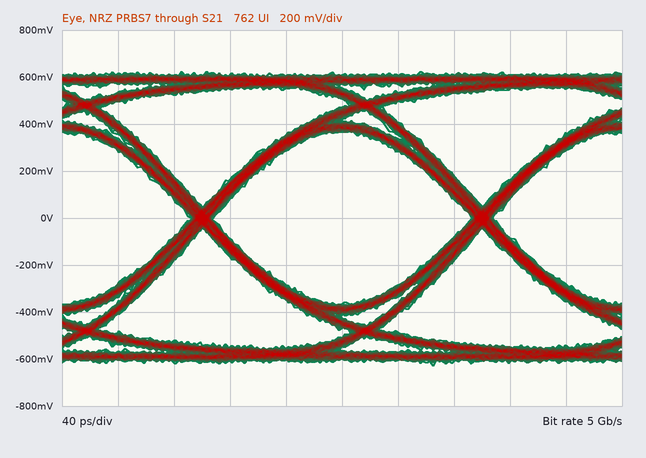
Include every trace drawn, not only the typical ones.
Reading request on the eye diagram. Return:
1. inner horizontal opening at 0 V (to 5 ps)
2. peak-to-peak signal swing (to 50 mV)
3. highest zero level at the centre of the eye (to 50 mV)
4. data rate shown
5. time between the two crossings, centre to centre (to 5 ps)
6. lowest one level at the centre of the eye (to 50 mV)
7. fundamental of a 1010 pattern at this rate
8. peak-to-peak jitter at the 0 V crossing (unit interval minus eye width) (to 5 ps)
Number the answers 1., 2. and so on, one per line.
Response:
1. 185 ps
2. 1.25 V
3. -350 mV
4. 5 Gb/s
5. 200 ps
6. 350 mV
7. 2.5 GHz
8. 15 ps
